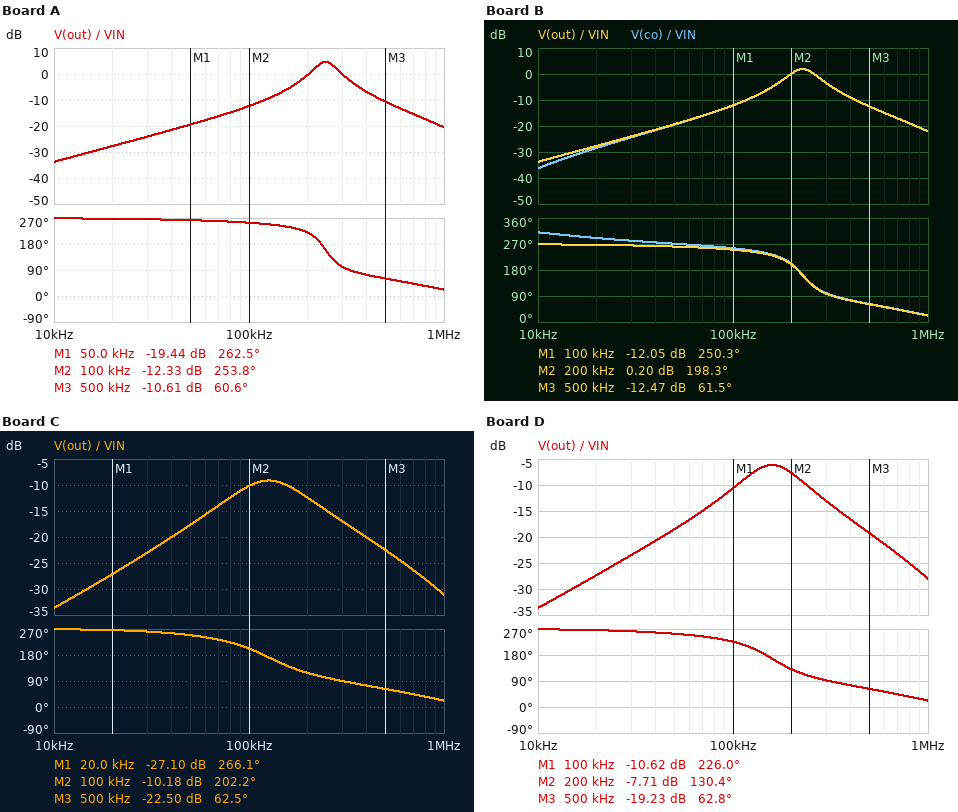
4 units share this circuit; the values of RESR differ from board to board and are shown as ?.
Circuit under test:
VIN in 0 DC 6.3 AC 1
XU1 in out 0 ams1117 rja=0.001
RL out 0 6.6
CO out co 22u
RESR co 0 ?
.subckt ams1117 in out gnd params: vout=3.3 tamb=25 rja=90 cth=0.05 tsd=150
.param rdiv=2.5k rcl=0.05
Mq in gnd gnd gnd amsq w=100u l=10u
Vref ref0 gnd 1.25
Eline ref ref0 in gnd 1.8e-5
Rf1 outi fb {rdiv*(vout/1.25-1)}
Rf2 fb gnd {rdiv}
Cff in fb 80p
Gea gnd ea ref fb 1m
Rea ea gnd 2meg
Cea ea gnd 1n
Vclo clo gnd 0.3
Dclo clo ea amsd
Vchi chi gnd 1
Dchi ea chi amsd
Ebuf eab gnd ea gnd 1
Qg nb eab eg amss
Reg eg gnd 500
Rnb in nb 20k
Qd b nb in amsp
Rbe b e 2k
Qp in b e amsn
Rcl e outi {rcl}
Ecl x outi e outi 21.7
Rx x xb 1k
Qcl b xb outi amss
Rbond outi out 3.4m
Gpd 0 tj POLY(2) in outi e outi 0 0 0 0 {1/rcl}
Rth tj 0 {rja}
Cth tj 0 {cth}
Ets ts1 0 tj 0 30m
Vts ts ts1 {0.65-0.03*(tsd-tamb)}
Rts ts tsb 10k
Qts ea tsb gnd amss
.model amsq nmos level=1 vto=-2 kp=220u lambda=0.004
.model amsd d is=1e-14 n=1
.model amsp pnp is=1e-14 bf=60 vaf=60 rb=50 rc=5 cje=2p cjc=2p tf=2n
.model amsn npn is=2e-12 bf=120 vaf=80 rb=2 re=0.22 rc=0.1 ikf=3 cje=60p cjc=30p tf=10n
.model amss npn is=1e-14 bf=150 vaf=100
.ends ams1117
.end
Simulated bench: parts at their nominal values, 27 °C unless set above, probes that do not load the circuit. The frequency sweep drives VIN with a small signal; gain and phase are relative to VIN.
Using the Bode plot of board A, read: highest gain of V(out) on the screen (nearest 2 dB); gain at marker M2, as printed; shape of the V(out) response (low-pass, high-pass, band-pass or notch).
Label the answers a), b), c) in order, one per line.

a) 4 dB
b) -12.33 dB
c) band-pass
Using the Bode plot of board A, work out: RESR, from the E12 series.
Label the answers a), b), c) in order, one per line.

a) 1 Ω
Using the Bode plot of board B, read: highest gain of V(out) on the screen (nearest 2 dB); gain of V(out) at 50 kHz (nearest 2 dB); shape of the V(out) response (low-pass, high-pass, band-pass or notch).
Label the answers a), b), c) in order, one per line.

a) 2 dB
b) -20 dB
c) band-pass
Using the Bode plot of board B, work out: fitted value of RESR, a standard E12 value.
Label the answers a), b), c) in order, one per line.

a) 0.82 Ω
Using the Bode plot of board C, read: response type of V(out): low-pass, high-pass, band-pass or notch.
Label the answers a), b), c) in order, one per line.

a) band-pass
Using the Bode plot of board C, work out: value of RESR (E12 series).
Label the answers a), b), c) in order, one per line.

a) 0.27 Ω
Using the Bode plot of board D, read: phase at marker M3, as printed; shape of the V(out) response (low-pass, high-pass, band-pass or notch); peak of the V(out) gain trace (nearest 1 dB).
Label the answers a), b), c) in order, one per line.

a) 62.8 deg
b) band-pass
c) -6 dB
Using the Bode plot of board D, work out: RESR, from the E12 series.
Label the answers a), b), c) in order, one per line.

a) 0.39 Ω
